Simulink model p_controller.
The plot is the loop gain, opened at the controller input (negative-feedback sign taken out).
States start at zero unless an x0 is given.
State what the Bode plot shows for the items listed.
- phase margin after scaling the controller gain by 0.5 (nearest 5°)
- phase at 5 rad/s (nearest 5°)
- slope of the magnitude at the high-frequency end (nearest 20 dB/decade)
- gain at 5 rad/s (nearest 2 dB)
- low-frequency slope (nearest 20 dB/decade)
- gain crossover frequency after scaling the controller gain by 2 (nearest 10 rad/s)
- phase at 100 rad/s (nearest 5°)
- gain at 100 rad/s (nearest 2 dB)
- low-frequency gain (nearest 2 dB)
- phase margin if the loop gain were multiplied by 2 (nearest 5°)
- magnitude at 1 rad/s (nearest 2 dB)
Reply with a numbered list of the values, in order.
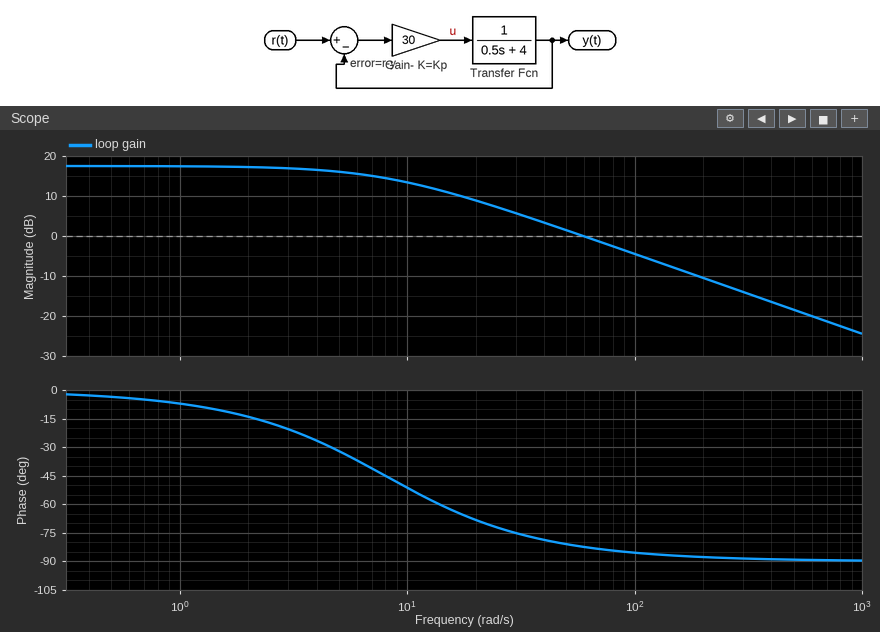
1. 105°
2. -30°
3. -20 dB/decade
4. 16 dB
5. 0 dB/decade
6. 120 rad/s
7. -85°
8. -4 dB
9. 18 dB
10. 95°
11. 18 dB
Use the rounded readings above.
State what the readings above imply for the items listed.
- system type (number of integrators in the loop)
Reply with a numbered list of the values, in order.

1. 0
